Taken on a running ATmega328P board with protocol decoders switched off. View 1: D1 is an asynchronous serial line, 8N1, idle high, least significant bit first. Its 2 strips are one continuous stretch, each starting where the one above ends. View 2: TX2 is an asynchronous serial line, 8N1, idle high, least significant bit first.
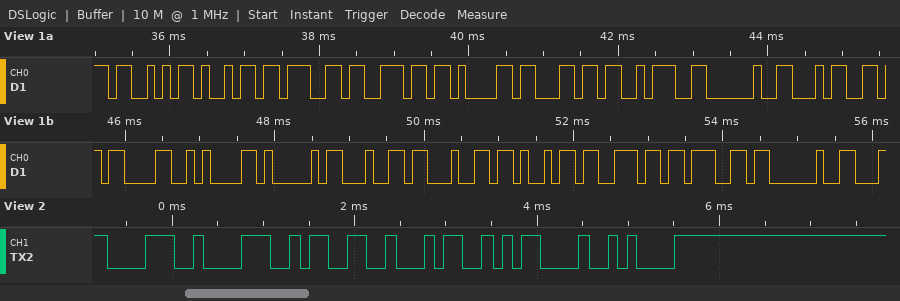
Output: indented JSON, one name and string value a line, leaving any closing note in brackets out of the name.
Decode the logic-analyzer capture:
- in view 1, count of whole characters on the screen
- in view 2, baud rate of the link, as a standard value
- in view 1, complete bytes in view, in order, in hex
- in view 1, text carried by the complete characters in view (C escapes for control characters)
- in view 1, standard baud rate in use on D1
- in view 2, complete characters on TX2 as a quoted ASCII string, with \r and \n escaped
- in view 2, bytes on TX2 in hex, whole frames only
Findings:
{
  "in view 1, count of whole characters on the screen": "18",
  "in view 2, baud rate of the link, as a standard value": "9600 baud",
  "in view 1, complete bytes in view, in order, in hex": "53 69 67 6E 61 6C 3A 20 34 0D 0A 41 64 64 69 6E 67 20",
  "in view 1, text carried by the complete characters in view": "\"Signal: 4\\r\\nAdding \"",
  "in view 1, standard baud rate in use on D1": "9600 baud",
  "in view 2, complete characters on TX2 as a quoted ASCII string, with \\r and \\n escaped": "\"8834\\r\\n\"",
  "in view 2, bytes on TX2 in hex, whole frames only": "0x38 0x38 0x33 0x34 0x0D 0x0A"
}
